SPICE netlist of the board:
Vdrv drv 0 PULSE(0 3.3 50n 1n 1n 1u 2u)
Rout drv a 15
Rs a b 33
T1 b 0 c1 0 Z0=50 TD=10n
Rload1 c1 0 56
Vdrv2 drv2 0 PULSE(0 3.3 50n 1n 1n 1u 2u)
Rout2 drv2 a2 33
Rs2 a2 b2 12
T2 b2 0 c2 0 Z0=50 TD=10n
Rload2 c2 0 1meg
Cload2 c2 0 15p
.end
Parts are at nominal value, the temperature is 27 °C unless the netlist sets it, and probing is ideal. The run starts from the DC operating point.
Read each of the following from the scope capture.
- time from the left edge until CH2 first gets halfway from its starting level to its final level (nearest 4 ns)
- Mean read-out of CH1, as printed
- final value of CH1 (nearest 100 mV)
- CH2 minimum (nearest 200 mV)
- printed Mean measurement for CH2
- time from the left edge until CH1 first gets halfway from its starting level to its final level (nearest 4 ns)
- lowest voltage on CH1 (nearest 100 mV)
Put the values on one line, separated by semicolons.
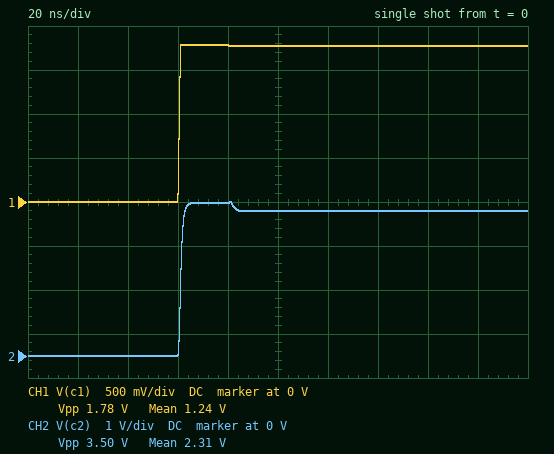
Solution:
60 ns; 1.24 V; 1.8 V; 0 V; 2.31 V; 60 ns; 0 V
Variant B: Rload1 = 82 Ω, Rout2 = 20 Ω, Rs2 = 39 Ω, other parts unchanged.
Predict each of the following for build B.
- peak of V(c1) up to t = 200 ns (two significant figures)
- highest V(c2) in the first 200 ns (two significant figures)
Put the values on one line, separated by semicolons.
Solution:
2.1 V; 3.3 V
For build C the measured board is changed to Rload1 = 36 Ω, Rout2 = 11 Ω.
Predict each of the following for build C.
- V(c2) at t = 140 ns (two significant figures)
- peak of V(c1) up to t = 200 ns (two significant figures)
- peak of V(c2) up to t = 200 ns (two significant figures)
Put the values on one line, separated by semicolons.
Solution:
3.2 V; 1.4 V; 4.7 V
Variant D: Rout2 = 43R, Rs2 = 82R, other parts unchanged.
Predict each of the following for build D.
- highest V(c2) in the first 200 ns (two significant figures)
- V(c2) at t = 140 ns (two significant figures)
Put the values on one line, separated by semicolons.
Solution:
3.3 V; 3.2 V
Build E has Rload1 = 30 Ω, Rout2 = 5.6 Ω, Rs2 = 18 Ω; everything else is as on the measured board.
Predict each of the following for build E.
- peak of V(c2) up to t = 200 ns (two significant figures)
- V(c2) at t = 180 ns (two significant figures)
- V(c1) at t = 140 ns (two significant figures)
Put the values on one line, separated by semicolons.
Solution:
4.7 V; 3.3 V; 1.3 V
